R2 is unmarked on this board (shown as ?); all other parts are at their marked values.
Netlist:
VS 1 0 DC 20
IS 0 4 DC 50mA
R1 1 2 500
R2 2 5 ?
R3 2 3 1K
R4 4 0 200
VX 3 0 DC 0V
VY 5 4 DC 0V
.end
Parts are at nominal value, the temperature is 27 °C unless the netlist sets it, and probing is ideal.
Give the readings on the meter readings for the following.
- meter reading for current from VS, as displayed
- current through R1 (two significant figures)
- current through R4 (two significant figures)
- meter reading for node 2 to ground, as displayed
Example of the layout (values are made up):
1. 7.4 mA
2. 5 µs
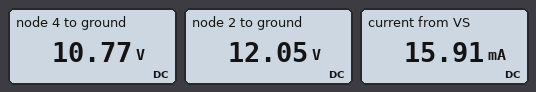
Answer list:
1. 15.91 mA
2. 16 mA
3. 54 mA
4. 12.05 V
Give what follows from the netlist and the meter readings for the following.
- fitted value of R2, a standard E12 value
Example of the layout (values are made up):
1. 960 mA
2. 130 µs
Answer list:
1. 330 Ω
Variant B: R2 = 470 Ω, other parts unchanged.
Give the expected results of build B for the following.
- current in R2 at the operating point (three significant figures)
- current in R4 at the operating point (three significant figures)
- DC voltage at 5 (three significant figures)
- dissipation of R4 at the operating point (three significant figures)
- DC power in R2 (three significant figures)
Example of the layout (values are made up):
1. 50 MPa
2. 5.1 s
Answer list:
1. 3.32 mA
2. 53.3 mA
3. 10.7 V
4. 569 mW
5. 5.19 mW
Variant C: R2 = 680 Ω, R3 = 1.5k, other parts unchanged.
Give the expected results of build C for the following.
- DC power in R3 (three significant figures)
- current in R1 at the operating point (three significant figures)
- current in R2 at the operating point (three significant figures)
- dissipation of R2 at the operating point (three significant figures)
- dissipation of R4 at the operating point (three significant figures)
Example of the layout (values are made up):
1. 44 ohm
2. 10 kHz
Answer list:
1. 122 mW
2. 13.0 mA
3. 3.98 mA
4. 10.8 mW
5. 583 mW
